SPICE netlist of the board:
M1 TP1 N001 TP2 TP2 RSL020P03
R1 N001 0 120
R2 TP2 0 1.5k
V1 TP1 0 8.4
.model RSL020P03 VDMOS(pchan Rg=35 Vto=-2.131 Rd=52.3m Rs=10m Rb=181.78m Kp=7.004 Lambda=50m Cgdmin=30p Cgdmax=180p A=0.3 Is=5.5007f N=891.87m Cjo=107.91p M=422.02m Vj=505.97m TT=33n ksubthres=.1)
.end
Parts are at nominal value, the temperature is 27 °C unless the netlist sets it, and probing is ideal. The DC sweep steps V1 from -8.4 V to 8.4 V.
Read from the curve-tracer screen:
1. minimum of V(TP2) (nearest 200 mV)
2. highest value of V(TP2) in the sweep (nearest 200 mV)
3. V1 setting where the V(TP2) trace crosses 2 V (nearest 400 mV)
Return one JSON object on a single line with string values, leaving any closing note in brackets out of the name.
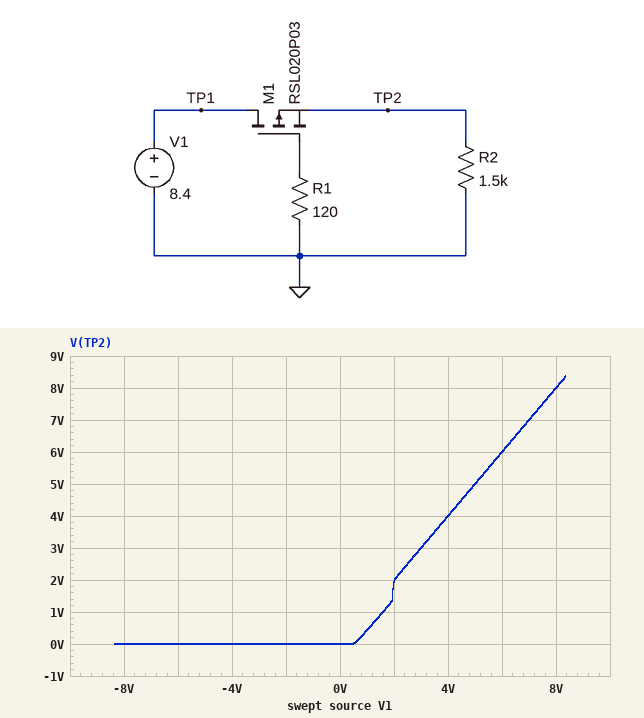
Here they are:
{"minimum of V(TP2)": "0 V", "highest value of V(TP2) in the sweep": "8.4 V", "V1 setting where the V(TP2) trace crosses 2 V": "2.0 V"}
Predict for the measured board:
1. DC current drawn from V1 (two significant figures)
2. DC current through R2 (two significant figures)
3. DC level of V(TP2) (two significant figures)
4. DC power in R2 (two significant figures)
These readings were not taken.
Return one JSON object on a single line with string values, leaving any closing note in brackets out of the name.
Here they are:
{"DC current drawn from V1": "5.6 mA", "DC current through R2": "5.6 mA", "DC level of V(TP2)": "8.4 V", "DC power in R2": "47 mW"}
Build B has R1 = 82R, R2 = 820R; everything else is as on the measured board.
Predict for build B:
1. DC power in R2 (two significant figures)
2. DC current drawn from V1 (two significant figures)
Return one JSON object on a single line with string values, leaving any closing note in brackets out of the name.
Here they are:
{"DC power in R2": "86 mW", "DC current drawn from V1": "10 mA"}
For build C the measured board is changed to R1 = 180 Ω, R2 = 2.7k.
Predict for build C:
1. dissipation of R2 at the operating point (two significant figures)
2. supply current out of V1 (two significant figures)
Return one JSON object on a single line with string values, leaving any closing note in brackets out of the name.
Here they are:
{"dissipation of R2 at the operating point": "26 mW", "supply current out of V1": "3.1 mA"}
